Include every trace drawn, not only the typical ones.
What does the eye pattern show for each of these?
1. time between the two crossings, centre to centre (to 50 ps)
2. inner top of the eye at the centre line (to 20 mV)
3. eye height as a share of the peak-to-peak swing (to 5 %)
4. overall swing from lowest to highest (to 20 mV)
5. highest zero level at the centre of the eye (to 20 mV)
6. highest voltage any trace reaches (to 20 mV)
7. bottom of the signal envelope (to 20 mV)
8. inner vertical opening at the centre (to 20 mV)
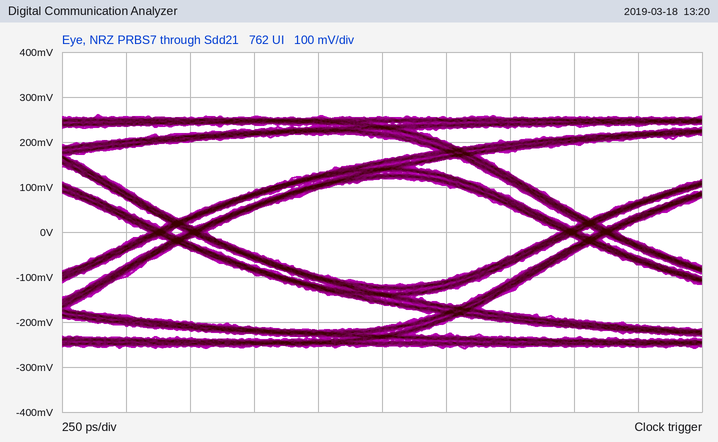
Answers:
1.60 ns
120 mV
45 %
520 mV
-120 mV
260 mV
-260 mV
240 mV
